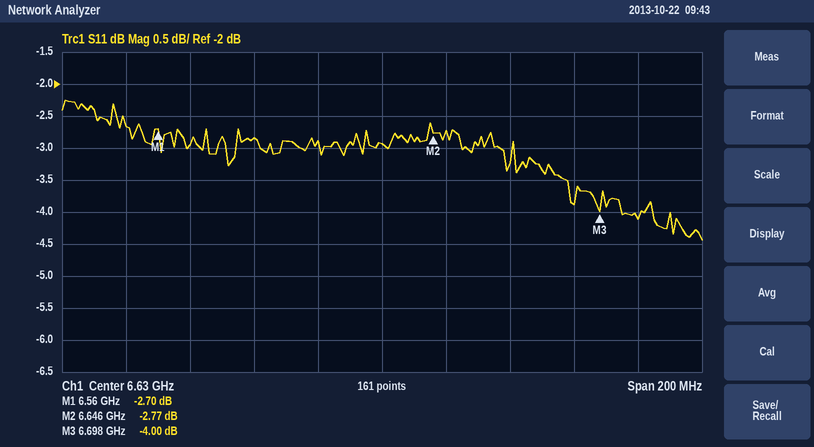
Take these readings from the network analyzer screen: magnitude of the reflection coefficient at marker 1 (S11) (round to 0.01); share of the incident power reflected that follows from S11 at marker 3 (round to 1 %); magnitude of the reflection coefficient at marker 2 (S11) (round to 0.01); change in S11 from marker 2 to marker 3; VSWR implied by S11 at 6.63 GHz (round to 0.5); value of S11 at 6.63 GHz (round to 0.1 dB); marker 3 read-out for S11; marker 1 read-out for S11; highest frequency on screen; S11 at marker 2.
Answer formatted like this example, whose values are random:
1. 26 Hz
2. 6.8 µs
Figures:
1. 0.73
2. 40 %
3. 0.73
4. -1.23 dB
5. 6.0
6. -2.9 dB
7. -4.00 dB
8. -2.70 dB
9. 6.73 GHz
10. -2.77 dB
